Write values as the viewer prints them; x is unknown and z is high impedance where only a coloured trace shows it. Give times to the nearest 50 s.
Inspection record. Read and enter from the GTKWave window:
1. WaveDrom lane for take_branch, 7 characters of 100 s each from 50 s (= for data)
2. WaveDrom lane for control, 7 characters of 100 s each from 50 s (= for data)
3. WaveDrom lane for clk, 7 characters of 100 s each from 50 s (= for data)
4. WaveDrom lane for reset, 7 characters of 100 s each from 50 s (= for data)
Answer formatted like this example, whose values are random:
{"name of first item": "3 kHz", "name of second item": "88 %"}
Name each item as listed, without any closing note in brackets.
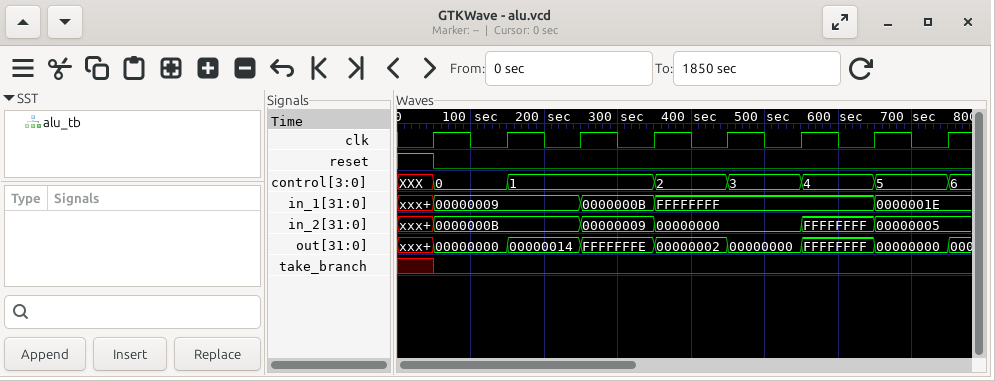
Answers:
{"WaveDrom lane for take_branch, 7 characters of 100 s each from 50 s": "{name: 'take_branch', wave: '0......'}", "WaveDrom lane for control, 7 characters of 100 s each from 50 s": "{name: 'control', wave: '==.====', data: '0 1 2 3 4 5'}", "WaveDrom lane for clk, 7 characters of 100 s each from 50 s": "{name: 'clk', wave: 'p......'}", "WaveDrom lane for reset, 7 characters of 100 s each from 50 s": "{name: 'reset', wave: '0......'}"}
